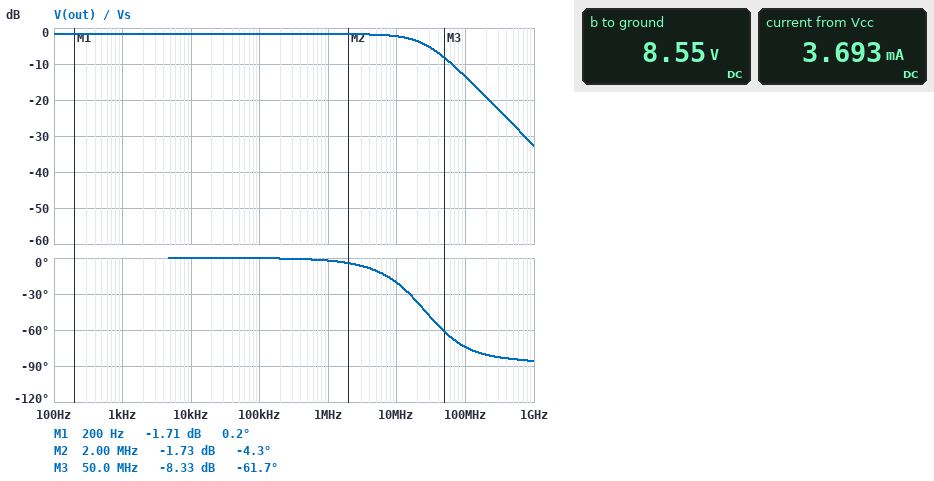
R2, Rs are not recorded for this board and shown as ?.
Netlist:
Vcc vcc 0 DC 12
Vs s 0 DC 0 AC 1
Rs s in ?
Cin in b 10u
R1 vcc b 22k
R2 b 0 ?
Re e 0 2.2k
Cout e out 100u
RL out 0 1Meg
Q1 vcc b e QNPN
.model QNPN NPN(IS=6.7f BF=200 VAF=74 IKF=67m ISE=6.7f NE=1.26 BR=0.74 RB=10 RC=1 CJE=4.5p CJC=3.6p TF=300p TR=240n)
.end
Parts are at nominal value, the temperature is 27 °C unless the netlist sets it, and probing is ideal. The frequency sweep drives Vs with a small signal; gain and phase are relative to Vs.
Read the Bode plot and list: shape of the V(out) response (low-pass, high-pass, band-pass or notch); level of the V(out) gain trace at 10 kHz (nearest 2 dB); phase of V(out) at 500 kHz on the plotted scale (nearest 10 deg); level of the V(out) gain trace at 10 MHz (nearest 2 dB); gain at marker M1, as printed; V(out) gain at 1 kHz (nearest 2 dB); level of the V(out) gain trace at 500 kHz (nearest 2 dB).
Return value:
low-pass
-2 dB
0 deg
-2 dB
-1.71 dB
-2 dB
-2 dB
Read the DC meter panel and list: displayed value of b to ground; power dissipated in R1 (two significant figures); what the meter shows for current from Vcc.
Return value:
8.55 V
540 µW
3.693 mA
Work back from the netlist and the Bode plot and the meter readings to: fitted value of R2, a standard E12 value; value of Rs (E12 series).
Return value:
68 kΩ
3.3 kΩ
